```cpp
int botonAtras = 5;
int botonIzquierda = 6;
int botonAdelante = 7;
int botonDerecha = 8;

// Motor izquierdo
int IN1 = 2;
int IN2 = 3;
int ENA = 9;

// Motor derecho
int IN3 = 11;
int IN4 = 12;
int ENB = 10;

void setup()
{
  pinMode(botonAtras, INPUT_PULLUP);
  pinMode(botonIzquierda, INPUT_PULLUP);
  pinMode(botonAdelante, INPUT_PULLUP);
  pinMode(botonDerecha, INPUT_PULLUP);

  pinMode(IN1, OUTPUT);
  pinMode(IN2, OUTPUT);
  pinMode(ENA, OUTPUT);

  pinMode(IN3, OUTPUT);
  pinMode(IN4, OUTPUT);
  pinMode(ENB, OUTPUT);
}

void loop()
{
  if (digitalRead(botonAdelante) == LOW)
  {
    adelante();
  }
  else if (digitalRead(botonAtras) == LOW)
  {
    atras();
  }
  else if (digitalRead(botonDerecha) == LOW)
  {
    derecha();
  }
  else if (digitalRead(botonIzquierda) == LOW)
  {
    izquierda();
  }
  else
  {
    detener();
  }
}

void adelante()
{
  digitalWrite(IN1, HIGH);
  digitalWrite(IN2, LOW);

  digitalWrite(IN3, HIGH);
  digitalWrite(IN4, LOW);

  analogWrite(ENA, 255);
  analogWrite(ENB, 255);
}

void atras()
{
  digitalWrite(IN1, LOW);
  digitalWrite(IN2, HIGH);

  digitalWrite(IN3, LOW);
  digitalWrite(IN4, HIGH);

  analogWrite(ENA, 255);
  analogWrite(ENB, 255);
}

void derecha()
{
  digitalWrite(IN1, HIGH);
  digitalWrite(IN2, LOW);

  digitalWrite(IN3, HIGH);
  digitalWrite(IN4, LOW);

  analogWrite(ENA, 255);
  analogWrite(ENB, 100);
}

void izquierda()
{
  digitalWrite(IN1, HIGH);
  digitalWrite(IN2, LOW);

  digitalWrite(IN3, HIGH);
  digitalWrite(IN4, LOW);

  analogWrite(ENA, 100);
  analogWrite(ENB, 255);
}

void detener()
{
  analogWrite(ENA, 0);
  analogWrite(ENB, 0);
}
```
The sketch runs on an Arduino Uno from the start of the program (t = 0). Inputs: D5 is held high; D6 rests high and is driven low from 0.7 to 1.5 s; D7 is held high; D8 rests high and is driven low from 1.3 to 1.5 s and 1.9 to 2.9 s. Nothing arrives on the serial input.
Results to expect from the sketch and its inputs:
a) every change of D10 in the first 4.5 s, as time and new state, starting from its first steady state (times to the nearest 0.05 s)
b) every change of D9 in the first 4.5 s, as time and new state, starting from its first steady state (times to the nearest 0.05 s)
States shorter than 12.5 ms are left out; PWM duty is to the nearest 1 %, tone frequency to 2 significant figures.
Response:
0 s low; 0.7 s high; 1.3 s PWM 39 %; 1.5 s low; 1.9 s PWM 39 %; 2.9 s low
0 s low; 0.7 s PWM 39 %; 1.3 s high; 1.5 s low; 1.9 s high; 2.9 s low
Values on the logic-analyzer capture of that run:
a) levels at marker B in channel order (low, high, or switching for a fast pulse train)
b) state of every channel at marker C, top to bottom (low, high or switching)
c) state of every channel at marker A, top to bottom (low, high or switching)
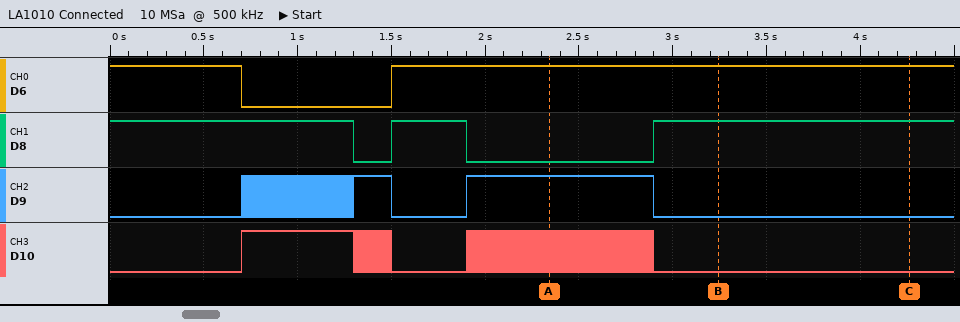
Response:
D6 high, D8 high, D9 low, D10 low
D6 high, D8 high, D9 low, D10 low
D6 high, D8 low, D9 high, D10 switching
